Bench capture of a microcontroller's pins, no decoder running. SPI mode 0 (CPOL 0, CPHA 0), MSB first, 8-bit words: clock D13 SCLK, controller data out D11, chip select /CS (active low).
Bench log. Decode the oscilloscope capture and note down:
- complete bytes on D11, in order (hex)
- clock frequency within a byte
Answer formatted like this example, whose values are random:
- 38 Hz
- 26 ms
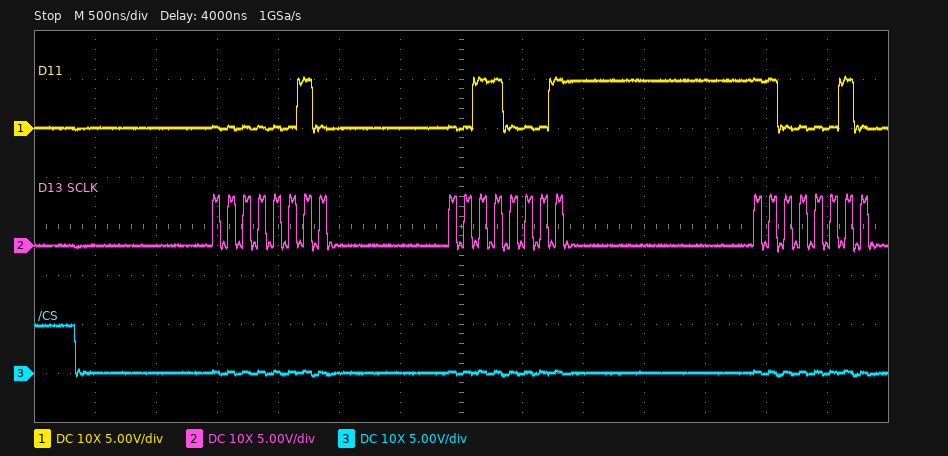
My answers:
- 0x02 0x31 0xC2
- 8 MHz
